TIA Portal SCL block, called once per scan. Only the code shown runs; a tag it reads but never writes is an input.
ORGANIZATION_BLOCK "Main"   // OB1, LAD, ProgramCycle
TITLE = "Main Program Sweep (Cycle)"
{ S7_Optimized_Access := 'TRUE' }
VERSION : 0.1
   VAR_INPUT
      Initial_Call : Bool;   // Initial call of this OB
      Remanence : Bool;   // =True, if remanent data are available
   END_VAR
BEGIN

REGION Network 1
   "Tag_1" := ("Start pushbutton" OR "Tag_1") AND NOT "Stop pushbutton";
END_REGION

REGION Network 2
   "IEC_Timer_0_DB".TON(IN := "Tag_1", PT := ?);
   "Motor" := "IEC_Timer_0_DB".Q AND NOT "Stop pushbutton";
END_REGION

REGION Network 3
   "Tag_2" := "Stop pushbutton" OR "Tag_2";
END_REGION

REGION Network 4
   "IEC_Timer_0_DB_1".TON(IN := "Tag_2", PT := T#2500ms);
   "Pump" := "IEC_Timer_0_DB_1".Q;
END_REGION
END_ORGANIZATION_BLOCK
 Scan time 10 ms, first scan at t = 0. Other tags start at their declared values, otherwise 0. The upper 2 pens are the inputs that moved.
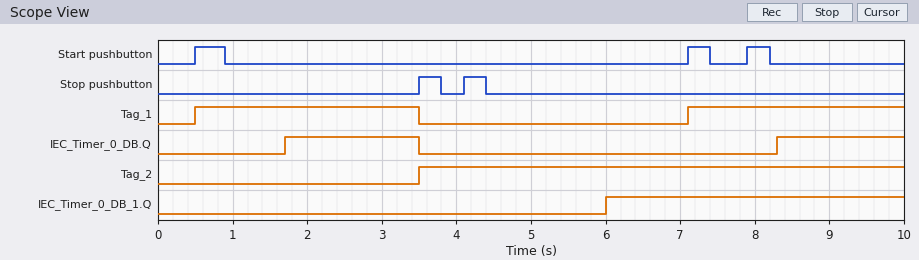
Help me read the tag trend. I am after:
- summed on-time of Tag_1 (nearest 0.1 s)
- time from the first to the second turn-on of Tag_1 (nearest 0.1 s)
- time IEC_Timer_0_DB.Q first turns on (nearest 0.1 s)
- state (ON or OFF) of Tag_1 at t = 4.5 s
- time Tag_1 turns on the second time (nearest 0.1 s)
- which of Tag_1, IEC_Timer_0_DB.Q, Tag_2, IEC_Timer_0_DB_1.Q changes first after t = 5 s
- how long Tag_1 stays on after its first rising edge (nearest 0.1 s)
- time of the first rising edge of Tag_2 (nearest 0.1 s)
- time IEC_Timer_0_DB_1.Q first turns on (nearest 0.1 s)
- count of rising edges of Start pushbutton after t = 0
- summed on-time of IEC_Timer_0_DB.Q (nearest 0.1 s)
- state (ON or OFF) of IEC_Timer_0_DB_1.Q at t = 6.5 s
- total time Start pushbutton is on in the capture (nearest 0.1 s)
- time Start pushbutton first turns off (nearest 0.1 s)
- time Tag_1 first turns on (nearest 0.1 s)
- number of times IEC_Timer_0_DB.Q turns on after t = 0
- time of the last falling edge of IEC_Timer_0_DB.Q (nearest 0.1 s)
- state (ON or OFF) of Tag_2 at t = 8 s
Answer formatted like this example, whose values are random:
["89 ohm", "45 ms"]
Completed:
["5.9 s", "6.6 s", "1.7 s", "OFF", "7.1 s", "IEC_Timer_0_DB_1.Q", "3.0 s", "3.5 s", "6.0 s", "3", "3.5 s", "ON", "1.0 s", "0.9 s", "0.5 s", "2", "3.5 s", "ON"]
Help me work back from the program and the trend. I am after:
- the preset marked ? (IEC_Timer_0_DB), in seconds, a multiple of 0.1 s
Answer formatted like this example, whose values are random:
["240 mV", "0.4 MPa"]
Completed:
["1.2 s"]
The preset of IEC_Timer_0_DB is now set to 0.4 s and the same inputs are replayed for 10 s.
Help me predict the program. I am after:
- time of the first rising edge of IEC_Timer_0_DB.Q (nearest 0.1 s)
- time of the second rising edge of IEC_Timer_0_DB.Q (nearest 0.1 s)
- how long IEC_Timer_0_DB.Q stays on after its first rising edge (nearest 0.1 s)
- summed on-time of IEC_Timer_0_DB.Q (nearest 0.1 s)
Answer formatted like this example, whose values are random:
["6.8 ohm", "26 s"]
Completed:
["0.9 s", "7.5 s", "2.6 s", "5.1 s"]
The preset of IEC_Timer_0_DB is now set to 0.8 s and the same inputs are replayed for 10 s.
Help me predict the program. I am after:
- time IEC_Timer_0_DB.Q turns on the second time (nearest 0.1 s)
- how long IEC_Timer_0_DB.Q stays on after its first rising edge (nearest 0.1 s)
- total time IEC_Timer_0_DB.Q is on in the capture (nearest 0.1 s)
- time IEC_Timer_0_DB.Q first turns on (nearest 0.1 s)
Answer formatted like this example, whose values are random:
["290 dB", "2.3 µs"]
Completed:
["7.9 s", "2.2 s", "4.3 s", "1.3 s"]
